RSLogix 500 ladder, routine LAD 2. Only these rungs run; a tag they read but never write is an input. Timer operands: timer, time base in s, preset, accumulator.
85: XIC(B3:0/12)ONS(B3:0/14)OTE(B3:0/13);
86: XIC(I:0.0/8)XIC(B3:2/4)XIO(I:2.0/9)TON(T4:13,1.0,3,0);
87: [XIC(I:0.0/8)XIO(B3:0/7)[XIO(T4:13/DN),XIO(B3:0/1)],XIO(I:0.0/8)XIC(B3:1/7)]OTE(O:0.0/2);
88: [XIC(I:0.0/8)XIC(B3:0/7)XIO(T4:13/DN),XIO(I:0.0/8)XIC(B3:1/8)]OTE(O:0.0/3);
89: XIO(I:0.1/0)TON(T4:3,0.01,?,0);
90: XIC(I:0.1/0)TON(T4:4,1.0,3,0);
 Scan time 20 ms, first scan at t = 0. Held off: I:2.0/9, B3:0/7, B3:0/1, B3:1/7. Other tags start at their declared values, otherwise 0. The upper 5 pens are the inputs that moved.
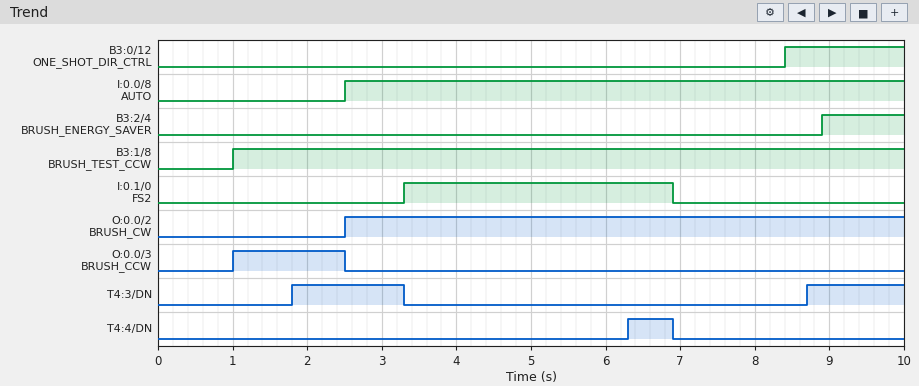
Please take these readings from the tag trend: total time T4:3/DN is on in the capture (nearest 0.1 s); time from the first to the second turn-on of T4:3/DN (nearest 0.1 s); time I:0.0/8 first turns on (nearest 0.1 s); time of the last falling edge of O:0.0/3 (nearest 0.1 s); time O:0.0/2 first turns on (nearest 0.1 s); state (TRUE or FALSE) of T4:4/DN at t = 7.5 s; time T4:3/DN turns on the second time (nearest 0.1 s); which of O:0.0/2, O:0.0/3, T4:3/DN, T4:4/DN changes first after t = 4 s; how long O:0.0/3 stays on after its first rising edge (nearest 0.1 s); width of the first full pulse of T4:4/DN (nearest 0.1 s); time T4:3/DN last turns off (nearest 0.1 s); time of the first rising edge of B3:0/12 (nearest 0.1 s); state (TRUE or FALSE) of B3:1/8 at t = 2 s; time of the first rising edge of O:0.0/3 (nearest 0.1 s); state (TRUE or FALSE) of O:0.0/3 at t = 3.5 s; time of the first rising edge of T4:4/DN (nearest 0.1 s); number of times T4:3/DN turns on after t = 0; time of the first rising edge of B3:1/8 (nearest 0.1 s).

2.8 s
6.9 s
2.5 s
2.5 s
2.5 s
FALSE
8.7 s
T4:4/DN
1.5 s
0.6 s
3.3 s
8.4 s
TRUE
1.0 s
FALSE
6.3 s
2
1.0 s
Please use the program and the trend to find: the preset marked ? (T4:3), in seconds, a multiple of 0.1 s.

1.8 s
